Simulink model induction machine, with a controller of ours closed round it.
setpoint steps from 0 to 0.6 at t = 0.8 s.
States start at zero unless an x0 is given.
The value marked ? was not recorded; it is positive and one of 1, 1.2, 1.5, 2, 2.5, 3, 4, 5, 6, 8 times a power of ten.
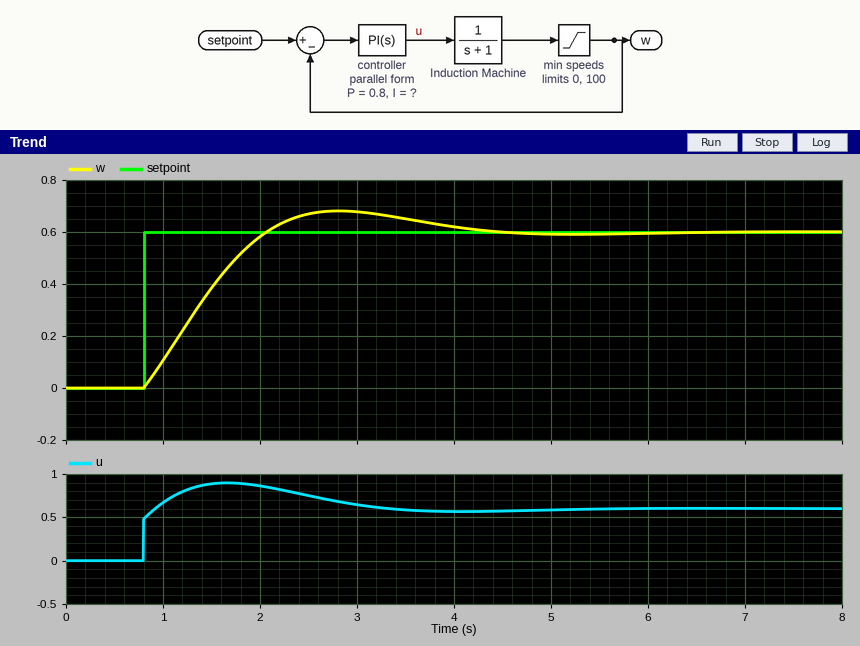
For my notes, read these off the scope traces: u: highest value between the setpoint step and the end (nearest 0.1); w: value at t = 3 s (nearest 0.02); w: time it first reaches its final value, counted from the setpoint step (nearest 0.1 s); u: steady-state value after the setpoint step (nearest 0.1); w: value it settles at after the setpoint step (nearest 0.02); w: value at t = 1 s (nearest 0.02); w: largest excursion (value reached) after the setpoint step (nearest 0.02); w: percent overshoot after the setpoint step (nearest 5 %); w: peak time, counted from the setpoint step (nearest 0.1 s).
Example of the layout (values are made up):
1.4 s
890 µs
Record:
0.9
0.68
1.3 s
0.6
0.60
0.10
0.68
15 %
2.0 s
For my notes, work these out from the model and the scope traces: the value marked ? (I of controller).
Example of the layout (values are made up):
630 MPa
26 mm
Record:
2.5
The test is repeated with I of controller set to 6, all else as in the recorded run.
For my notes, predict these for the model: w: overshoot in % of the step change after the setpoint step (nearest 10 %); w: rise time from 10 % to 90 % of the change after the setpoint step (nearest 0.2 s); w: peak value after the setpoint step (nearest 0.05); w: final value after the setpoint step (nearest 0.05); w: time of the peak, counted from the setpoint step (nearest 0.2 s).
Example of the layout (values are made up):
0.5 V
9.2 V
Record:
30 %
0.6 s
0.80
0.60
1.2 s
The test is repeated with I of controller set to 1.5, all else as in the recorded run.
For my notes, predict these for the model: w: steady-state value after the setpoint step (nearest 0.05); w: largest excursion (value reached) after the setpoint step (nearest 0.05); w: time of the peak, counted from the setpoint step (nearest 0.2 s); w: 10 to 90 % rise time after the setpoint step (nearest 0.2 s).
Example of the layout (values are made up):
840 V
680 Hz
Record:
0.60
0.65
3.0 s
1.4 s
